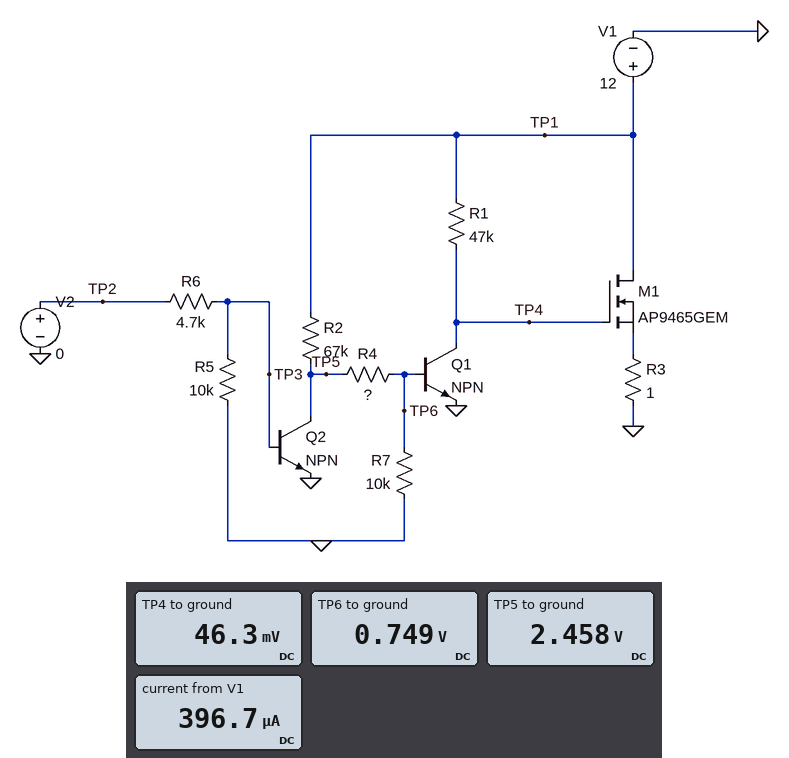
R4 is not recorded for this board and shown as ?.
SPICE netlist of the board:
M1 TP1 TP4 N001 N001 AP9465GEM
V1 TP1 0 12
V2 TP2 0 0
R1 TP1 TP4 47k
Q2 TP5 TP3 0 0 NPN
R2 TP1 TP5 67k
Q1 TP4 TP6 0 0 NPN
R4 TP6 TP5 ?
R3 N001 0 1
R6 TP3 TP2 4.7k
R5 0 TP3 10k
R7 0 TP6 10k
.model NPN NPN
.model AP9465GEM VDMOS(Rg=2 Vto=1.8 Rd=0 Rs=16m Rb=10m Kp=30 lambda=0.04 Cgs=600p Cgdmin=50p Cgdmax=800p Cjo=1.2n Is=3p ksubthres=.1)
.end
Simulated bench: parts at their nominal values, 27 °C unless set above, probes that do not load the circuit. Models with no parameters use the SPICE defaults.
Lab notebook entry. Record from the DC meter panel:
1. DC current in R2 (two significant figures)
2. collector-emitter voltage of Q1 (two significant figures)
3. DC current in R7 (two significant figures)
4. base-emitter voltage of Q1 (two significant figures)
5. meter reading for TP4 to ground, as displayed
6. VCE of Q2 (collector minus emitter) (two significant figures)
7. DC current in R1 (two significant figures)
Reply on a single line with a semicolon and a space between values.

140 µA; 46 mV; 75 µA; 750 mV; 46.3 mV; 2.5 V; 250 µA
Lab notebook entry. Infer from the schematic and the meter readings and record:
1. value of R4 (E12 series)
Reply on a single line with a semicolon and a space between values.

12 kΩ
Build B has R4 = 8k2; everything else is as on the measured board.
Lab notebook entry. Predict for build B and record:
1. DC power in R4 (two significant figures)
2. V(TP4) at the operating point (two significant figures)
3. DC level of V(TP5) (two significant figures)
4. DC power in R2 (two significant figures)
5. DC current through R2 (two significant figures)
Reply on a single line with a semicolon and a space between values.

180 µW; 45 mV; 2.0 V; 1.5 mW; 150 µA
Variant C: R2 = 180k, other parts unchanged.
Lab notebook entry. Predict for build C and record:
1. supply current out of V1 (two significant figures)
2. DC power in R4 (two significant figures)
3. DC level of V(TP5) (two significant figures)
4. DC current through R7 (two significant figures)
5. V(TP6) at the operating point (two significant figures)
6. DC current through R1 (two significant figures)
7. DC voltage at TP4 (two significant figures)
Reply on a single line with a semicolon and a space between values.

9.3 A; 42 µW; 1.3 V; 59 µA; 590 mV; 940 nA; 12 V
